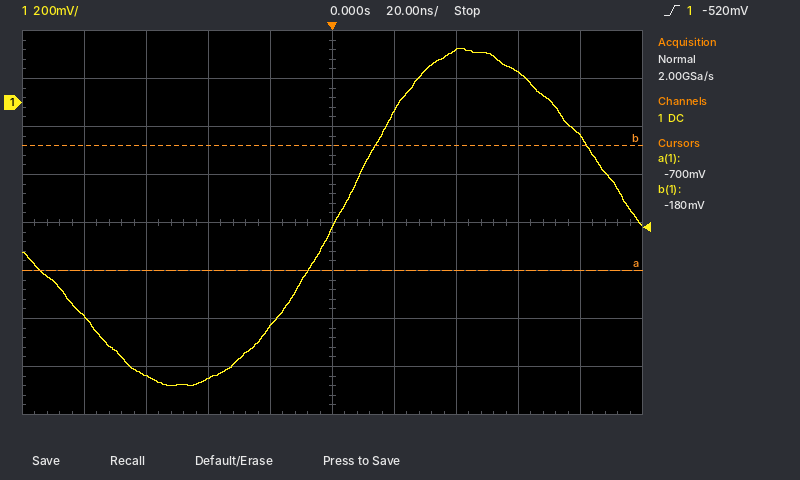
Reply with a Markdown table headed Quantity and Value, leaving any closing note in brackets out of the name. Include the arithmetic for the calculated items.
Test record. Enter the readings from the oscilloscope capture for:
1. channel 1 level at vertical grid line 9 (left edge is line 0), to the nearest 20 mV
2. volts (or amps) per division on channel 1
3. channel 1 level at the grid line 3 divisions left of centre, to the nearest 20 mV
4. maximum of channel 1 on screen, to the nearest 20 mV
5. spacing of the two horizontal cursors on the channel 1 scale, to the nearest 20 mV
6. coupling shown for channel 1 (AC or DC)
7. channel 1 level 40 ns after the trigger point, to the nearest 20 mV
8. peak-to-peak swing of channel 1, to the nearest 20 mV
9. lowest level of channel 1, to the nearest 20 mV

| Quantity | Value |
|---|---|
| channel 1 level at vertical grid line 9 (left edge is line 0), to the nearest 20 mV | -140 mV |
| volts (or amps) per division on channel 1 | 200 mV |
| channel 1 level at the grid line 3 divisions left of centre, to the nearest 20 mV | -1.14 V |
| maximum of channel 1 on screen, to the nearest 20 mV | 220 mV |
| spacing of the two horizontal cursors on the channel 1 scale, to the nearest 20 mV | 520 mV |
| coupling shown for channel 1 | DC |
| channel 1 level 40 ns after the trigger point, to the nearest 20 mV | 220 mV |
| peak-to-peak swing of channel 1, to the nearest 20 mV | 220 mV − (-1.18 V) = 1.40 V |
| lowest level of channel 1, to the nearest 20 mV | -1.18 V |
